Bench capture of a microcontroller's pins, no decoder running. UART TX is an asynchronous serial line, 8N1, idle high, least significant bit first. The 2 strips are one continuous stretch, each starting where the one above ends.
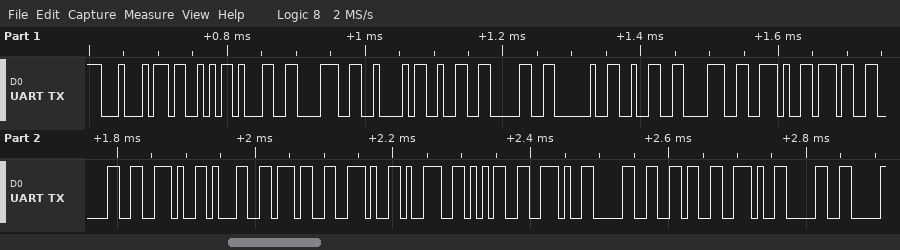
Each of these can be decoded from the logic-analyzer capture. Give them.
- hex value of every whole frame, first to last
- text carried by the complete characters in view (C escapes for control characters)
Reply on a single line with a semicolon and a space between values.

0x44 0x53 0x31 0x38 0x42 0x32 0x30 0x20 0x32 0x38 0x2E 0x37 0x30 0x2E 0x31 0x37 0x2E 0x39 0x35 0x2E 0x30 0x36 0x2E 0x30; "DS18B20 28.70.17.95.06.0"
